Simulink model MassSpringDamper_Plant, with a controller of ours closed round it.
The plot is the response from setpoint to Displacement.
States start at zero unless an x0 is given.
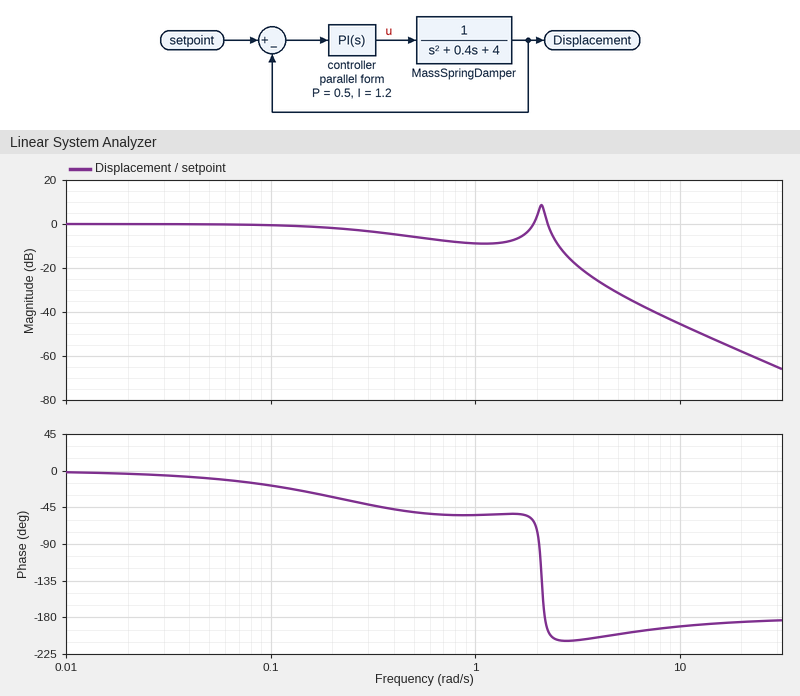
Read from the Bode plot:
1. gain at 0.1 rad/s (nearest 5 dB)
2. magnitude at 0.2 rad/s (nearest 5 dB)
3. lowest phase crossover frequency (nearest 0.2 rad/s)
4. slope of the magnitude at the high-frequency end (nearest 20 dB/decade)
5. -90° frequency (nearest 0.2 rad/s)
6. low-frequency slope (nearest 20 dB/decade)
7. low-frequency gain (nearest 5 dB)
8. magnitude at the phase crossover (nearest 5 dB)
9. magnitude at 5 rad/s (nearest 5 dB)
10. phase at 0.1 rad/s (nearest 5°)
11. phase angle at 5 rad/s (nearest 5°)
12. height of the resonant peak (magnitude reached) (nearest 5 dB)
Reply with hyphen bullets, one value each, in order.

- 0 dB
- 0 dB
- 2.2 rad/s
- -40 dB/decade
- 2.0 rad/s
- 0 dB/decade
- 0 dB
- 5 dB
- -30 dB
- -20°
- -200°
- 10 dB
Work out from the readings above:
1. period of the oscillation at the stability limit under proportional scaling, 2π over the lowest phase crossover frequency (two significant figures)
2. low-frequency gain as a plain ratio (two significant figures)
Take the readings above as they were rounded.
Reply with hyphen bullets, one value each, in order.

- 2.9 s
- 1.0
